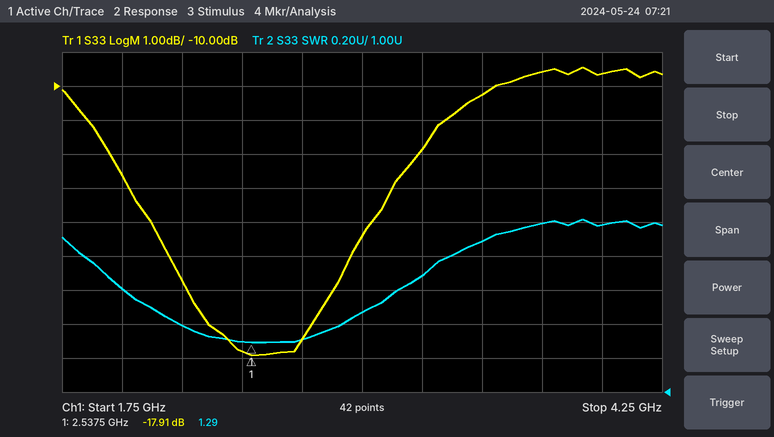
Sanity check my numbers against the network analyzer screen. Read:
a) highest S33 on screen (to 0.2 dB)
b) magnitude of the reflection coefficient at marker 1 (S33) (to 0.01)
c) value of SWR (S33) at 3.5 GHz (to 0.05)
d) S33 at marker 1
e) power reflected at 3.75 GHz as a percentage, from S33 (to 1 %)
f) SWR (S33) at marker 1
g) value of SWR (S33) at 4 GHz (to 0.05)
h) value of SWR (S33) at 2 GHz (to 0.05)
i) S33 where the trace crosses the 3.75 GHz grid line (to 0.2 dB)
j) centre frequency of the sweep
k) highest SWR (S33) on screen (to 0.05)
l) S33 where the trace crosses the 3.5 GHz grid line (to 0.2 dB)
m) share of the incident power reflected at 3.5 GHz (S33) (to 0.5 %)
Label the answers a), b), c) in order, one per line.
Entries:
a) -9.4 dB
b) 0.13
c) 1.90
d) -17.91 dB
e) 11 %
f) 1.29
g) 2.00
h) 1.60
i) -9.6 dB
j) 3 GHz
k) 2.00
l) -10.2 dB
m) 9.5 %
